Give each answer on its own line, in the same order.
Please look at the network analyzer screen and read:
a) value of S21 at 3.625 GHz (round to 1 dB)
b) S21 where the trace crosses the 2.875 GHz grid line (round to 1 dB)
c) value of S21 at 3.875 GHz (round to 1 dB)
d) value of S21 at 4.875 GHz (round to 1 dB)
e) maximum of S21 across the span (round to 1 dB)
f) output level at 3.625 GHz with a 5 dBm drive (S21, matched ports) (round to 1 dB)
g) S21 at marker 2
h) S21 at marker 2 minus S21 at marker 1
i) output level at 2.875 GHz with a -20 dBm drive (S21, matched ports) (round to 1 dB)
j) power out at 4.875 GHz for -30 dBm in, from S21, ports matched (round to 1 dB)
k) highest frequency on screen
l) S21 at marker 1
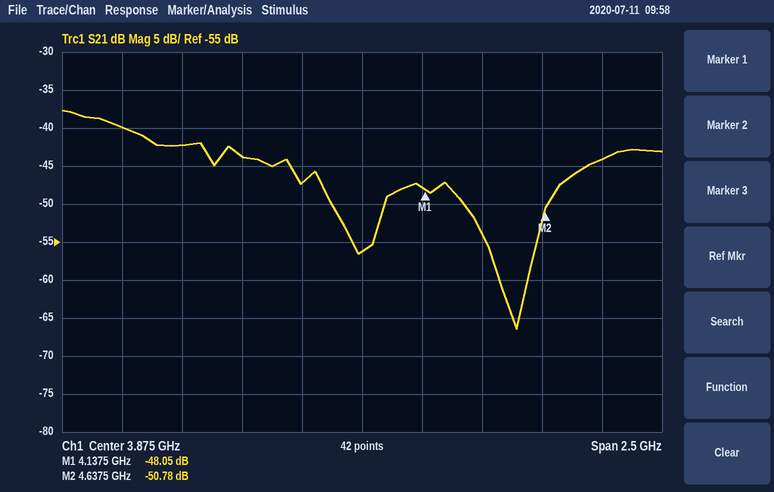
-47 dB
-40 dB
-56 dB
-44 dB
-38 dB
-42 dBm
-50.78 dB
-2.73 dB
-60 dBm
-74 dBm
5.125 GHz
-48.05 dB
